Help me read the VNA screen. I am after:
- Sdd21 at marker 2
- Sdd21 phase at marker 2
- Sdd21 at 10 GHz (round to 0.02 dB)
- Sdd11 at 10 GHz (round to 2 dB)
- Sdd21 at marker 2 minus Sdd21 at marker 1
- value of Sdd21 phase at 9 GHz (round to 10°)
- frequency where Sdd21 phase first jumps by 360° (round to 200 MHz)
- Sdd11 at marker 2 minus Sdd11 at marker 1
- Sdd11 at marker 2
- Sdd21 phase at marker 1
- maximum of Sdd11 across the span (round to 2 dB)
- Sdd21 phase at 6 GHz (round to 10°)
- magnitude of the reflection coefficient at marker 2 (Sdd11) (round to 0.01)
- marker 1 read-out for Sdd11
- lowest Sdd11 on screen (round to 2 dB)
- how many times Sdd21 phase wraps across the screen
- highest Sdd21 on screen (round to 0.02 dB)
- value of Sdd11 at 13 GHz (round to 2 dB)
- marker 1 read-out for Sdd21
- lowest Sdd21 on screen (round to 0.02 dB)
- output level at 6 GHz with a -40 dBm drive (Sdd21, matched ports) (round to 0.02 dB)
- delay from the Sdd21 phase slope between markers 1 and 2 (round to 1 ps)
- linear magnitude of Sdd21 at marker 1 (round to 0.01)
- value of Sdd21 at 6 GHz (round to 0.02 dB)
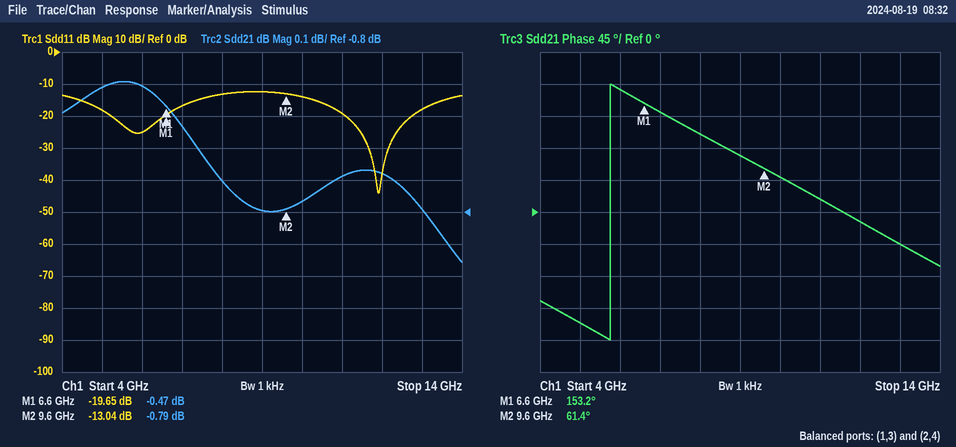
-0.79 dB
61.4°
-0.76 dB
-14 dB
-0.32 dB
80°
5.8 GHz
6.61 dB
-13.04 dB
153.2°
-12 dB
170°
0.22
-19.65 dB
-44 dB
1
-0.40 dB
-18 dB
-0.47 dB
-0.96 dB
-40.40 dBm
85 ps
0.95
-0.40 dB
